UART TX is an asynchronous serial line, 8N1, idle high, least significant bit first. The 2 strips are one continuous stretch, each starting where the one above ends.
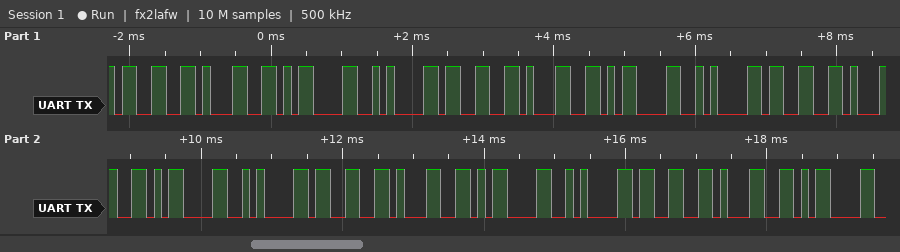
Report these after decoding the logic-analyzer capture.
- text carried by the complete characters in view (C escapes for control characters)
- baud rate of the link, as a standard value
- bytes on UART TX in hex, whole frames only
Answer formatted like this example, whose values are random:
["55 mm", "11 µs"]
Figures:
["\"31\\r\\n31\\r\\n31\\r\\n31\\r\\n31\\r\"", "9600 baud", "33 31 0D 0A 33 31 0D 0A 33 31 0D 0A 33 31 0D 0A 33 31 0D"]
